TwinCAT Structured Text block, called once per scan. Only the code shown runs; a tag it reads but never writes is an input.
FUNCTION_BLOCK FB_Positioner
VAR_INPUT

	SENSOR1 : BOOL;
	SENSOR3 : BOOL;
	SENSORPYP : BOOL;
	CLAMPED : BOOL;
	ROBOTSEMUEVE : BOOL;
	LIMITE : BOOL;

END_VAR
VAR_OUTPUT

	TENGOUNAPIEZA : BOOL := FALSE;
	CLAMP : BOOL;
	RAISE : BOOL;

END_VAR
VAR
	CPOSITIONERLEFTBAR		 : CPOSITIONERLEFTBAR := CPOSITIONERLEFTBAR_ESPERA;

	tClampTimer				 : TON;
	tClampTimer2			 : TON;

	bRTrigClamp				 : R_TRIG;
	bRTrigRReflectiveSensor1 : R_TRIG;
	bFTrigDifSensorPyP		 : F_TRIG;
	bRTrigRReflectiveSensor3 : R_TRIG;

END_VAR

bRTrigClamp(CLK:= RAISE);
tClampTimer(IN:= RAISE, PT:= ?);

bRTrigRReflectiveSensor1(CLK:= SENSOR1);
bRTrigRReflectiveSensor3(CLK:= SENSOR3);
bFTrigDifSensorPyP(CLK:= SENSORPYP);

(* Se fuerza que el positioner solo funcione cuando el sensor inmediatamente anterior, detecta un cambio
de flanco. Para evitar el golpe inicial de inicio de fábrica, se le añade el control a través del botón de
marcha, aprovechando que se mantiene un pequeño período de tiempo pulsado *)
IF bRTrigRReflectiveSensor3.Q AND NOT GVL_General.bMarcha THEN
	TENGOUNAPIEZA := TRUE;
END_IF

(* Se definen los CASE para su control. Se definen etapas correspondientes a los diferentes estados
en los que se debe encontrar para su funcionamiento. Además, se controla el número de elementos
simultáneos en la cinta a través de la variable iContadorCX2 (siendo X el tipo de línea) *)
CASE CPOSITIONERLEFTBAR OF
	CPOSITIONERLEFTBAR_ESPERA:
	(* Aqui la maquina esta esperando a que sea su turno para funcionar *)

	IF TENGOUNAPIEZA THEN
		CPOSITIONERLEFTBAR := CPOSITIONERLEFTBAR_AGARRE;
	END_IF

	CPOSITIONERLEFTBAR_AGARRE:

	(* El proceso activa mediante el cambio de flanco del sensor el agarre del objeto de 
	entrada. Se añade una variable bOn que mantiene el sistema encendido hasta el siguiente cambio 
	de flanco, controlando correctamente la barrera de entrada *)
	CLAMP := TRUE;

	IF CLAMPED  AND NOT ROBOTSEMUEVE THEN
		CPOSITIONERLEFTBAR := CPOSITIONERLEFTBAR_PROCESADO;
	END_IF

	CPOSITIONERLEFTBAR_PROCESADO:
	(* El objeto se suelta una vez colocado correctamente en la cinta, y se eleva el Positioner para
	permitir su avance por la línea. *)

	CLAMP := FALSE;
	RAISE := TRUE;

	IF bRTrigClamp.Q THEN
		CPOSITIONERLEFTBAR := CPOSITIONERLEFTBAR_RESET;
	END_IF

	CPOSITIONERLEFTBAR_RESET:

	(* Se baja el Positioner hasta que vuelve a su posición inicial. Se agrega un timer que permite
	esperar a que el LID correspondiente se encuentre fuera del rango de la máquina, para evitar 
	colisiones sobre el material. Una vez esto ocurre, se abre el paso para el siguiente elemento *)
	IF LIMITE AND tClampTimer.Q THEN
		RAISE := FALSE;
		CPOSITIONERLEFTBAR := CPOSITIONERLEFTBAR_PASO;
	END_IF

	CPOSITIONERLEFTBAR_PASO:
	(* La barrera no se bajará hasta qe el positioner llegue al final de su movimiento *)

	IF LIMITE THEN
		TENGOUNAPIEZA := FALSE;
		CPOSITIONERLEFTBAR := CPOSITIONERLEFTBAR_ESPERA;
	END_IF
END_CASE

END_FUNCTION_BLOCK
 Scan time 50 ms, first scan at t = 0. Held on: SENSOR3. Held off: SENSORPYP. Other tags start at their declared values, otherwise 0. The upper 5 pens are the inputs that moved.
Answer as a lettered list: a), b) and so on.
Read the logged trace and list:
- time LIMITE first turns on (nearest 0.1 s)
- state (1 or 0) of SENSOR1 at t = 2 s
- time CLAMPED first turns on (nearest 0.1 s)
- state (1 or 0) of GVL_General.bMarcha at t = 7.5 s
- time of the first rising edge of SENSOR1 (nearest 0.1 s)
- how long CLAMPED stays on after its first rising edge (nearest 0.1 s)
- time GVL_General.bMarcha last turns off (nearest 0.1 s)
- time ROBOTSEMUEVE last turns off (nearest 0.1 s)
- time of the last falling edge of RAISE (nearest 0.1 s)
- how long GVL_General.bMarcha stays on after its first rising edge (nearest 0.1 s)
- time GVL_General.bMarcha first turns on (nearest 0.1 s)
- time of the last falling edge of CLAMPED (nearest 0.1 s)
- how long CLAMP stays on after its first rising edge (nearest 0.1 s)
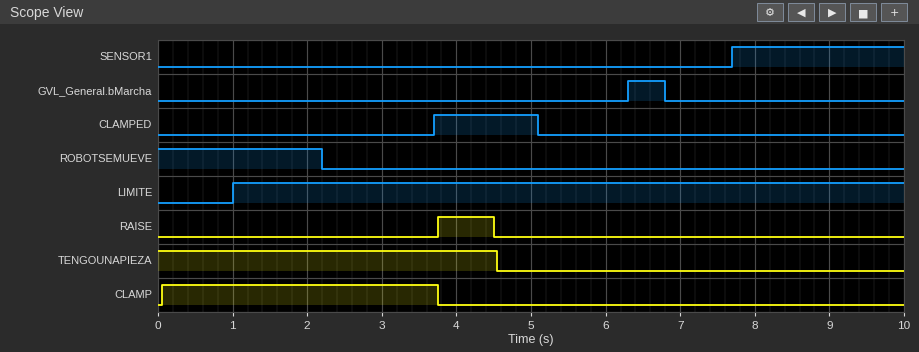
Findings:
a) 1.0 s
b) 0
c) 3.7 s
d) 0
e) 7.7 s
f) 1.4 s
g) 6.8 s
h) 2.2 s
i) 4.5 s
j) 0.5 s
k) 6.3 s
l) 5.1 s
m) 3.7 s
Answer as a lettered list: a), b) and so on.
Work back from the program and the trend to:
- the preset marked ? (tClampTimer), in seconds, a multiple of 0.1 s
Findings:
a) 0.7 s
